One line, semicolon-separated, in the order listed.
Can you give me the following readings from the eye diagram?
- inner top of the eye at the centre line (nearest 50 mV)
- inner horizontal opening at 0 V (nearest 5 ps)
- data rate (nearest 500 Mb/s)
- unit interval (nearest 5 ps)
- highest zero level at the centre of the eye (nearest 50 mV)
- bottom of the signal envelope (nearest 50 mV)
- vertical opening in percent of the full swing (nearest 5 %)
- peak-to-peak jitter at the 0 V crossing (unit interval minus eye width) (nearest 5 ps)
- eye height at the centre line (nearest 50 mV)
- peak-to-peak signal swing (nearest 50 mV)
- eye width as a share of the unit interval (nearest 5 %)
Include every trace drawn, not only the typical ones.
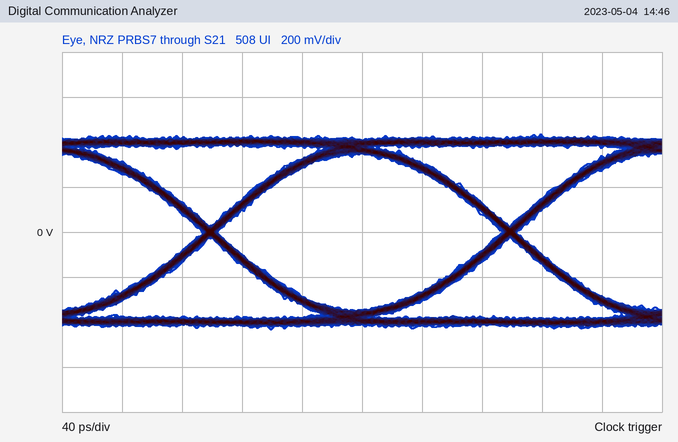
350 mV; 190 ps; 5.0 Gb/s; 200 ps; -350 mV; -450 mV; 80 %; 10 ps; 700 mV; 850 mV; 95 %
